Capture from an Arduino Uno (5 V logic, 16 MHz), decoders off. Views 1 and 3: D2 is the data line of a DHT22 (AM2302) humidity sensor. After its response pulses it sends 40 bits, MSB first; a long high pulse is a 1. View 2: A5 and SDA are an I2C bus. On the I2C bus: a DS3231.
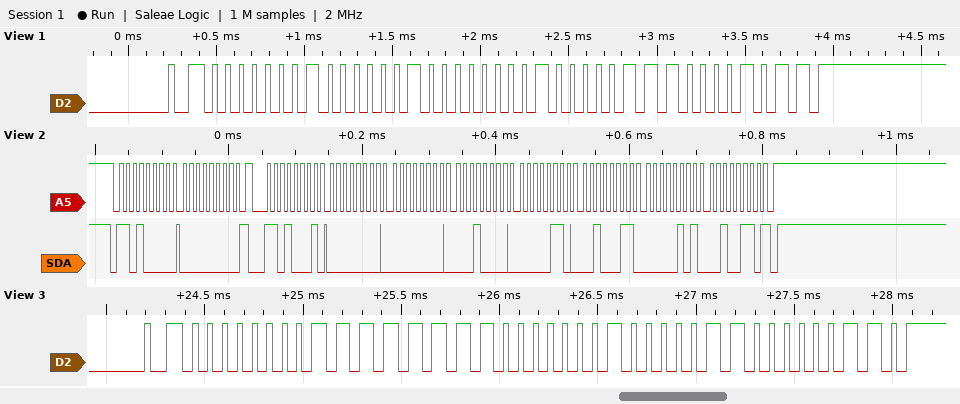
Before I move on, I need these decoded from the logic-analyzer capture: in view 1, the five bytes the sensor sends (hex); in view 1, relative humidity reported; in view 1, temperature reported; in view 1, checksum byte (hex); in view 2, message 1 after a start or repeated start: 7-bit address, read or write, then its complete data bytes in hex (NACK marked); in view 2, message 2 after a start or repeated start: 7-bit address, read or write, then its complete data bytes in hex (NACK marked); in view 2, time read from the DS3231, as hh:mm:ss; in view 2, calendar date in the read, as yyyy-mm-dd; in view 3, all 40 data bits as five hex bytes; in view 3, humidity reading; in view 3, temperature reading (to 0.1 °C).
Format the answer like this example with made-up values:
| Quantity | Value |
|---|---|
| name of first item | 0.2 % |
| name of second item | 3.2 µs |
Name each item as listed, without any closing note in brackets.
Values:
| Quantity | Value |
|---|---|
| in view 1, the five bytes the sensor sends | 01 02 01 07 0B |
| in view 1, relative humidity reported | 25.8 % |
| in view 1, temperature reported | 26.3 °C |
| in view 1, checksum byte | 0x0B |
| in view 2, message 1 after a start or repeated start: 7-bit address, read or write, then its complete data bytes in hex | 0x68 write: 00 |
| in view 2, message 2 after a start or repeated start: 7-bit address, read or write, then its complete data bytes in hex | 0x68 read: 00 00 10 06 23 05 26 NACK |
| in view 2, time read from the DS3231, as hh:mm:ss | 10:00:00 |
| in view 2, calendar date in the read, as yyyy-mm-dd | 2026-05-23 |
| in view 3, all 40 data bits as five hex bytes | 00 FF 01 06 06 |
| in view 3, humidity reading | 25.5 % |
| in view 3, temperature reading | 26.2 °C |
